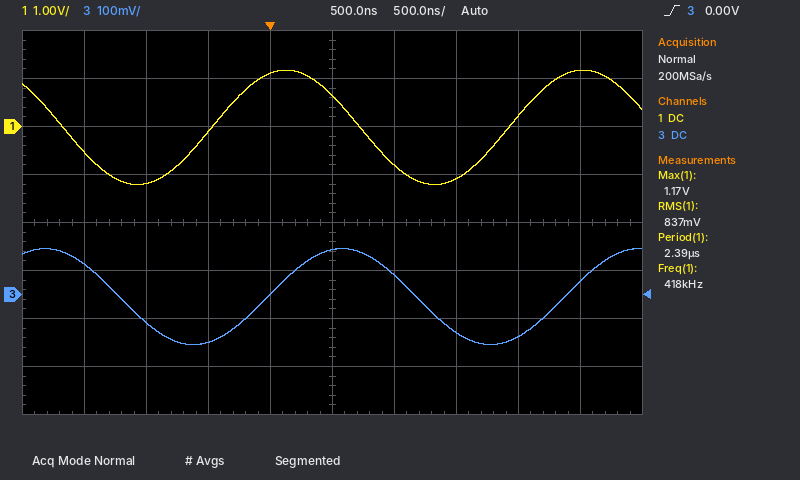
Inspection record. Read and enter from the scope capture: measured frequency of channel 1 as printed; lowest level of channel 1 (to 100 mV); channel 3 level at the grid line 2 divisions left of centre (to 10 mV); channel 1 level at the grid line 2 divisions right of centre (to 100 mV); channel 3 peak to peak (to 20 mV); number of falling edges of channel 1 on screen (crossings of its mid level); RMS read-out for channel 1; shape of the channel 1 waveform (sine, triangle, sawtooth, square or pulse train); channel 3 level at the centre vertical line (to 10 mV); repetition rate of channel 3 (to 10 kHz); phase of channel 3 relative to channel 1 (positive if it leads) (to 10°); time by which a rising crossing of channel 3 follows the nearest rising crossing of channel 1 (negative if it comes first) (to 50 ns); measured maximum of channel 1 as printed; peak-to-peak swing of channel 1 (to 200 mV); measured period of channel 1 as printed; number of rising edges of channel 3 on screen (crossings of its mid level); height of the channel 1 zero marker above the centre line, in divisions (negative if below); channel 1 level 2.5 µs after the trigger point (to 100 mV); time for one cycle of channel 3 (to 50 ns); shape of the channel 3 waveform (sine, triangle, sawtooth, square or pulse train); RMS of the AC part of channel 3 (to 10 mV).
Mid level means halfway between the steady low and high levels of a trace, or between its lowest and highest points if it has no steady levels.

418 kHz
-1.2 V
-100 mV
-1.1 V
200 mV
2
837 mV
sine
90 mV
420 kHz
-70°
+450 ns
1.17 V
2.4 V
2.39 µs
2
+2.0 div
1.2 V
2.40 µs
sine
70 mV
